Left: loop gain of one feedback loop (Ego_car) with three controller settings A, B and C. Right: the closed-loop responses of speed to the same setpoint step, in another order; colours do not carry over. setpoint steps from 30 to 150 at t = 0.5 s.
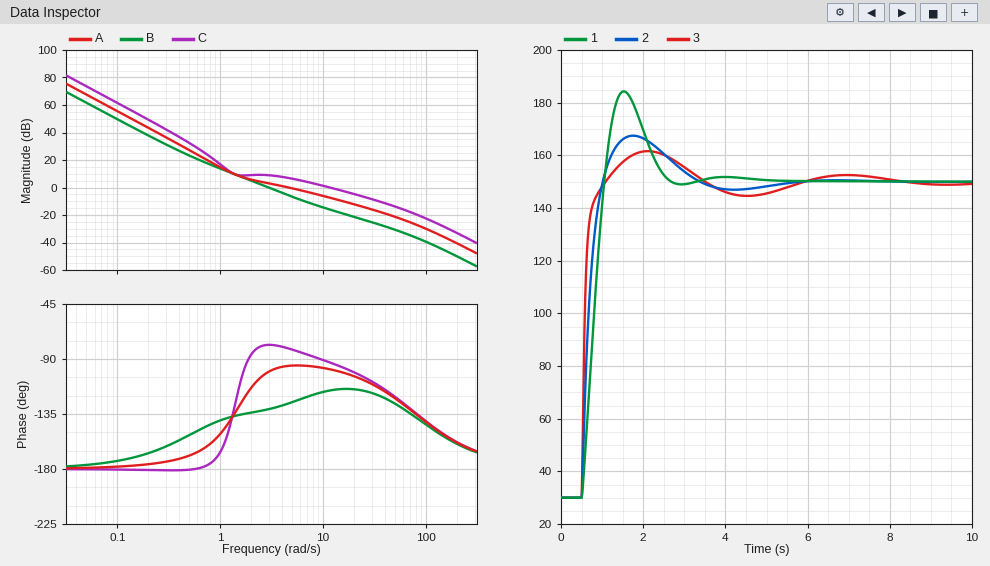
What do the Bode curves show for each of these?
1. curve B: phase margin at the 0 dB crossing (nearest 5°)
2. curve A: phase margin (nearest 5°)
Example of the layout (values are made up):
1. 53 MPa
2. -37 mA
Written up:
1. 50°
2. 85°
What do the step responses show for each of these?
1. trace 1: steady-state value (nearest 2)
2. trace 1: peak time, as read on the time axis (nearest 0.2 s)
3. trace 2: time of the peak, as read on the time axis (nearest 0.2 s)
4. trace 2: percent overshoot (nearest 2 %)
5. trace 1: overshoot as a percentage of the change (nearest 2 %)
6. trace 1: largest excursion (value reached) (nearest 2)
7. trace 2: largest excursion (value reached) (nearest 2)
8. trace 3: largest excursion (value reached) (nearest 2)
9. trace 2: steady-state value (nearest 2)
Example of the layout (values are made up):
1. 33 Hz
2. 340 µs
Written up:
1. 150
2. 1.6 s
3. 1.8 s
4. 14 %
5. 28 %
6. 184
7. 168
8. 162
9. 150
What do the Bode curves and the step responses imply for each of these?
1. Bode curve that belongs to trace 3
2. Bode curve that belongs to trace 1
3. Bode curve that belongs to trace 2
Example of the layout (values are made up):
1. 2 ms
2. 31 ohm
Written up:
1. C
2. B
3. A
